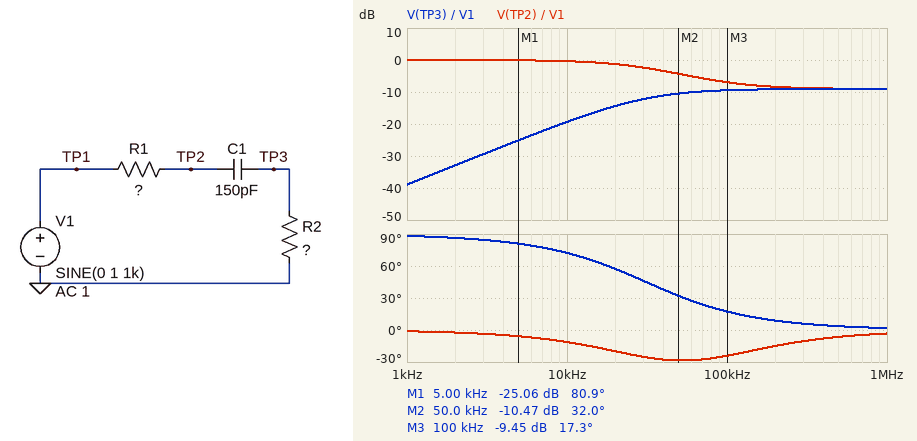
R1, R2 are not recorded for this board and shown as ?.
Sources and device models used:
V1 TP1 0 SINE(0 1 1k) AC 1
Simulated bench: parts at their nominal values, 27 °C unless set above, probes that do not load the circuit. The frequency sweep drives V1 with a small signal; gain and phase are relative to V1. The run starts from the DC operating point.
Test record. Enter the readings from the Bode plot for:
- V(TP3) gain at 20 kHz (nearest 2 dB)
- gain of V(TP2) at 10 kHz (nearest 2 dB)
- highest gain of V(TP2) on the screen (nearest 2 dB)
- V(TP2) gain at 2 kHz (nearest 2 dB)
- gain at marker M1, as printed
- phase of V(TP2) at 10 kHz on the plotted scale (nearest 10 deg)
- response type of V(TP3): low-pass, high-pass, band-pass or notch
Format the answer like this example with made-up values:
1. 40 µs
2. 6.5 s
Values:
1. -14 dB
2. 0 dB
3. 0 dB
4. 0 dB
5. -25.06 dB
6. -10 deg
7. high-pass
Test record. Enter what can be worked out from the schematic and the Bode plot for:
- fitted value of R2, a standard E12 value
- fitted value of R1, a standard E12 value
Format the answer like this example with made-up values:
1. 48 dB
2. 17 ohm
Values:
1. 12 kΩ
2. 22 kΩ
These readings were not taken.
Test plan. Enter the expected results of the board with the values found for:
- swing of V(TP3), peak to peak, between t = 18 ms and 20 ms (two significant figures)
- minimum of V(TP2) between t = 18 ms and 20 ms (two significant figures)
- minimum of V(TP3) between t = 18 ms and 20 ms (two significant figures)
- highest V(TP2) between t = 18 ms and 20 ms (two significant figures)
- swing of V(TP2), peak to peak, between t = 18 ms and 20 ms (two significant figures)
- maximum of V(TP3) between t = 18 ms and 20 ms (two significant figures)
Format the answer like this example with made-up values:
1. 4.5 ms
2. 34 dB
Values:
1. 23 mV
2. -1.0 V
3. -11 mV
4. 1.0 V
5. 2.0 V
6. 11 mV
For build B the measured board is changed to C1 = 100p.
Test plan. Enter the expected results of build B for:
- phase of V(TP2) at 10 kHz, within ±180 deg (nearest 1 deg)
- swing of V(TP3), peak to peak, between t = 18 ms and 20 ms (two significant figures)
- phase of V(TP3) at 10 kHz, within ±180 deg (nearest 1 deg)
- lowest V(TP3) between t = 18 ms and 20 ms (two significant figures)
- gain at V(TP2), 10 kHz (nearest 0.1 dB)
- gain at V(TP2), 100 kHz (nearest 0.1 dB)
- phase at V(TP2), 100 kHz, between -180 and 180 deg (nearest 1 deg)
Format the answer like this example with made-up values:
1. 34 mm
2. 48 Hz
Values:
1. -8 deg
2. 15 mV
3. 78 deg
4. -7.5 mV
5. -0.2 dB
6. -5.5 dB
7. -28 deg
